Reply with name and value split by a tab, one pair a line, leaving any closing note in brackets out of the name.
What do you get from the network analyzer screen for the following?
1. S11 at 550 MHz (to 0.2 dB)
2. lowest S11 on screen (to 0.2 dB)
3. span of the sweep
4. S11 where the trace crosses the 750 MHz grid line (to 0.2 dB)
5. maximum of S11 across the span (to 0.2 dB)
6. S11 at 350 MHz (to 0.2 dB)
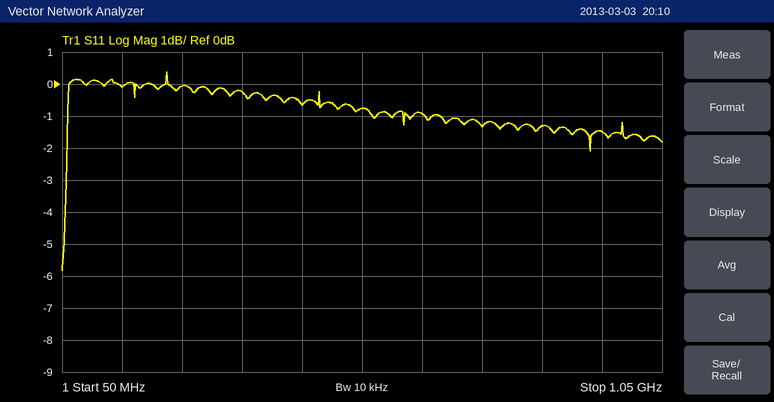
S11 at 550 MHz	-0.8 dB
lowest S11 on screen	-5.8 dB
span of the sweep	1 GHz
S11 where the trace crosses the 750 MHz grid line	-1.4 dB
maximum of S11 across the span	0.4 dB
S11 at 350 MHz	-0.2 dB
